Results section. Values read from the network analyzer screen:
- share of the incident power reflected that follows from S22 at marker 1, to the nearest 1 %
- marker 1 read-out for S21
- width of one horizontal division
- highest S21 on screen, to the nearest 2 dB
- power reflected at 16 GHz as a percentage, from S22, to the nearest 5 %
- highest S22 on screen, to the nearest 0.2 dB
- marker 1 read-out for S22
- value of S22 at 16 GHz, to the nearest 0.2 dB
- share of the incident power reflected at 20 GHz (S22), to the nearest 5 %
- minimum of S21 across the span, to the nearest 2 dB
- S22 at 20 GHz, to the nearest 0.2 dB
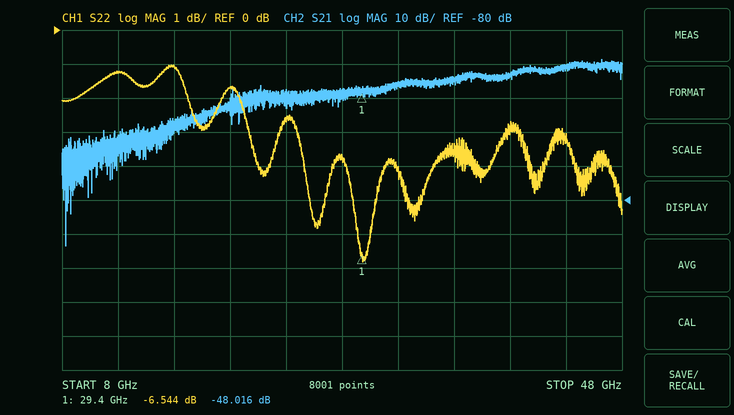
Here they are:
22 %
-48.016 dB
4 GHz
-38 dB
80 %
-1.0 dB
-6.544 dB
-1.0 dB
70 %
-94 dB
-1.6 dB
